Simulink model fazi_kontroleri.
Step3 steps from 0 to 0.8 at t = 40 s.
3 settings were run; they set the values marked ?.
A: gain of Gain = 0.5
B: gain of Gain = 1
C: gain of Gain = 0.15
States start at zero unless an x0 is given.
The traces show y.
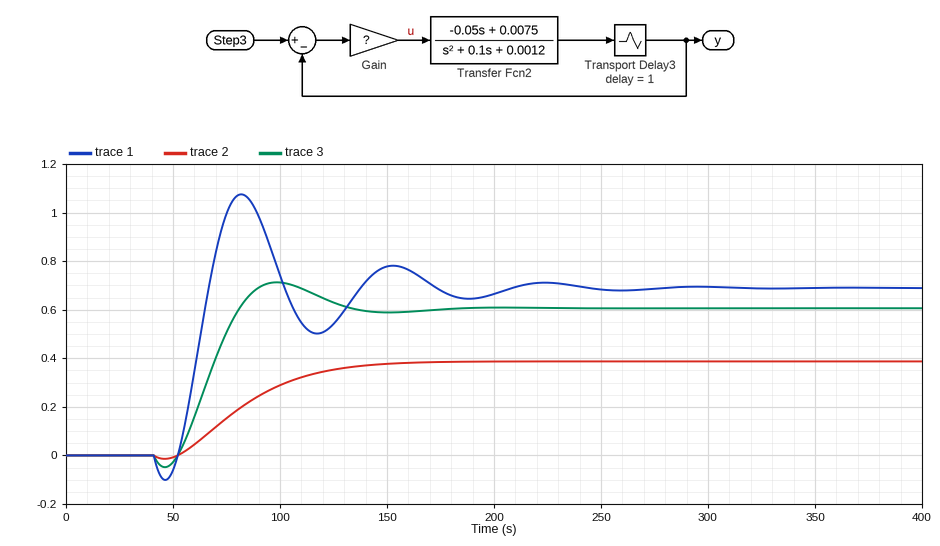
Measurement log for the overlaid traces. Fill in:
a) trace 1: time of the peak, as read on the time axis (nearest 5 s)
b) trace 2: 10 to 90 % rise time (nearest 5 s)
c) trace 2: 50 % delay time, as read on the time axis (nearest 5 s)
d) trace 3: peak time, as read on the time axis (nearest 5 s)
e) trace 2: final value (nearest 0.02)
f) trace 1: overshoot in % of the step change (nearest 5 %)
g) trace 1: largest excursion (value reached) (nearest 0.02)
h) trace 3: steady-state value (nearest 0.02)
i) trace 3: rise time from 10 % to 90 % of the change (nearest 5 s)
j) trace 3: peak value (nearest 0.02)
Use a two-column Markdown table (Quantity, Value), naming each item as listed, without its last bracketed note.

| Quantity | Value |
|---|---|
| trace 1: time of the peak, as read on the time axis | 80 s |
| trace 2: 10 to 90 % rise time | 65 s |
| trace 2: 50 % delay time, as read on the time axis | 80 s |
| trace 3: peak time, as read on the time axis | 100 s |
| trace 2: final value | 0.38 |
| trace 1: overshoot in % of the step change | 55 % |
| trace 1: largest excursion (value reached) | 1.08 |
| trace 3: steady-state value | 0.60 |
| trace 3: rise time from 10 % to 90 % of the change | 20 s |
| trace 3: peak value | 0.72 |
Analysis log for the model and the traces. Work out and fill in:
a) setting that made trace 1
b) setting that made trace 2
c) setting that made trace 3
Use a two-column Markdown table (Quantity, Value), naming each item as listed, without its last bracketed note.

| Quantity | Value |
|---|---|
| setting that made trace 1 | B |
| setting that made trace 2 | C |
| setting that made trace 3 | A |
